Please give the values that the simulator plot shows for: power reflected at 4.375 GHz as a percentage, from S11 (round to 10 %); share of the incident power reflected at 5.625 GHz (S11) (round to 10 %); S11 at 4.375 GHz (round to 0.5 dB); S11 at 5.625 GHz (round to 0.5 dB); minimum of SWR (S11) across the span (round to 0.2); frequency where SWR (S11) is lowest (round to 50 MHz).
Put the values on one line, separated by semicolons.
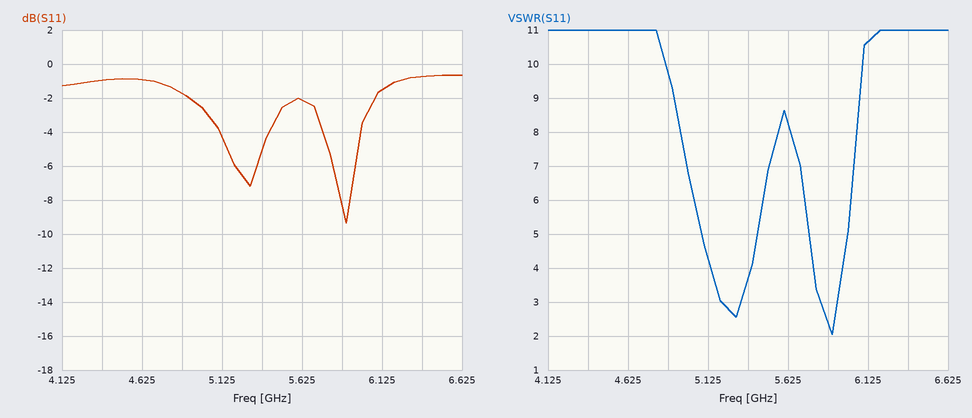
80 %; 60 %; -1.0 dB; -2.0 dB; 2.0; 5.90 GHz
